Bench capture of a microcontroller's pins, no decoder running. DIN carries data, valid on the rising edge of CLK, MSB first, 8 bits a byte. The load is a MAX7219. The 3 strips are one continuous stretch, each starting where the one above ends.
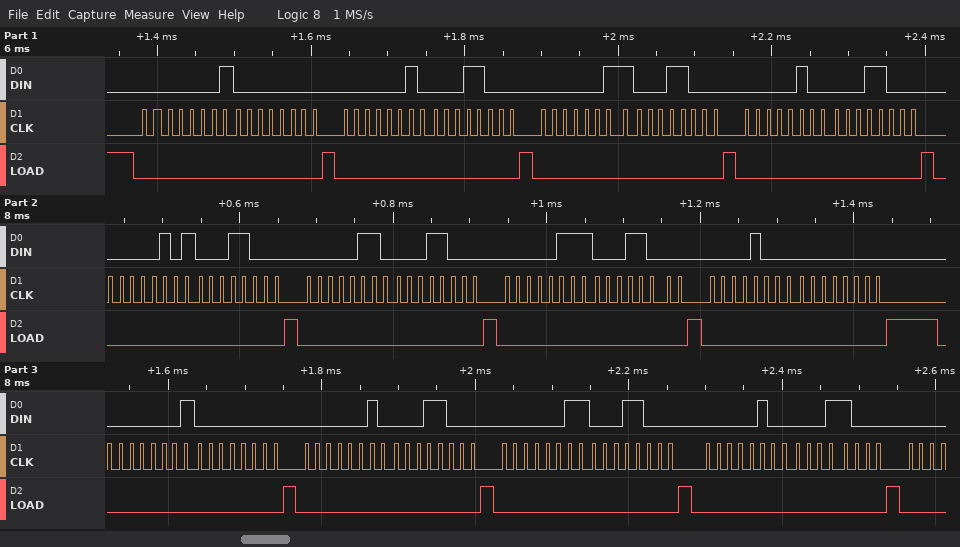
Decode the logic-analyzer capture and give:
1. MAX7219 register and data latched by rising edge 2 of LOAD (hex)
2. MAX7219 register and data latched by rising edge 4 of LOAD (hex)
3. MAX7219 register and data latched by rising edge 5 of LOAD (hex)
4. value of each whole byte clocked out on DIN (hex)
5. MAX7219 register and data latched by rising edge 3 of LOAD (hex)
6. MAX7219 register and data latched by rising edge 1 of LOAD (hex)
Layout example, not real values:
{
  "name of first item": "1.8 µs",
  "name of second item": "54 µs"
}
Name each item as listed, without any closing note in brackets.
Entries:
{
  "MAX7219 register and data latched by rising edge 2 of LOAD": "register 0x2, data 0x18",
  "MAX7219 register and data latched by rising edge 4 of LOAD": "register 0x4, data 0x18",
  "MAX7219 register and data latched by rising edge 5 of LOAD": "register 0x5, data 0x18",
  "value of each whole byte clocked out on DIN": "01 00 02 18 03 18 04 18 05 18 06 18 07 18 08 00 01 00 02 18 03 18 04 18",
  "MAX7219 register and data latched by rising edge 3 of LOAD": "register 0x3, data 0x18",
  "MAX7219 register and data latched by rising edge 1 of LOAD": "register 0x1, data 0x00"
}
